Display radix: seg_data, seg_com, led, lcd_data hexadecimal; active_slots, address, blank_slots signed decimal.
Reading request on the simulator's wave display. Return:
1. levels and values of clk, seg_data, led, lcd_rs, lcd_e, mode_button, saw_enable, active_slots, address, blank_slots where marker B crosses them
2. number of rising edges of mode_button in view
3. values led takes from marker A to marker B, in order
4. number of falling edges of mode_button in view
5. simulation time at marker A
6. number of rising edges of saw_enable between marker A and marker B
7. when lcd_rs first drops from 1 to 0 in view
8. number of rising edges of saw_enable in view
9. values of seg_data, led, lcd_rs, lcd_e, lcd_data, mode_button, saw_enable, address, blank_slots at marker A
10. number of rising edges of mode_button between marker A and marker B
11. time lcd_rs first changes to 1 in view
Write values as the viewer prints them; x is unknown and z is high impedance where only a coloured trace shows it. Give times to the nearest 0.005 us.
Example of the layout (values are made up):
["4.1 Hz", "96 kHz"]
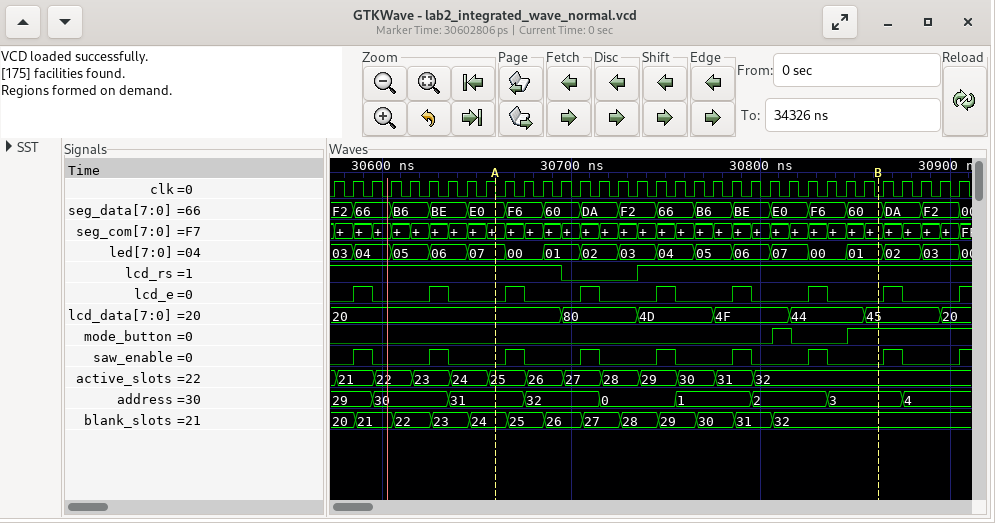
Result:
["clk=0, seg_data=60, led=01, lcd_rs=1, lcd_e=0, mode_button=1, saw_enable=0, active_slots=32, address=3, blank_slots=32", "2", "07, 00, 01, 02, 03, 04, 05, 06, 07, 00, 01", "1", "30.66 us", "5", "30.695 us", "9", "seg_data=E0, led=07, lcd_rs=1, lcd_e=0, lcd_data=20, mode_button=0, saw_enable=0, address=31, blank_slots=24", "2", "30.735 us"]
